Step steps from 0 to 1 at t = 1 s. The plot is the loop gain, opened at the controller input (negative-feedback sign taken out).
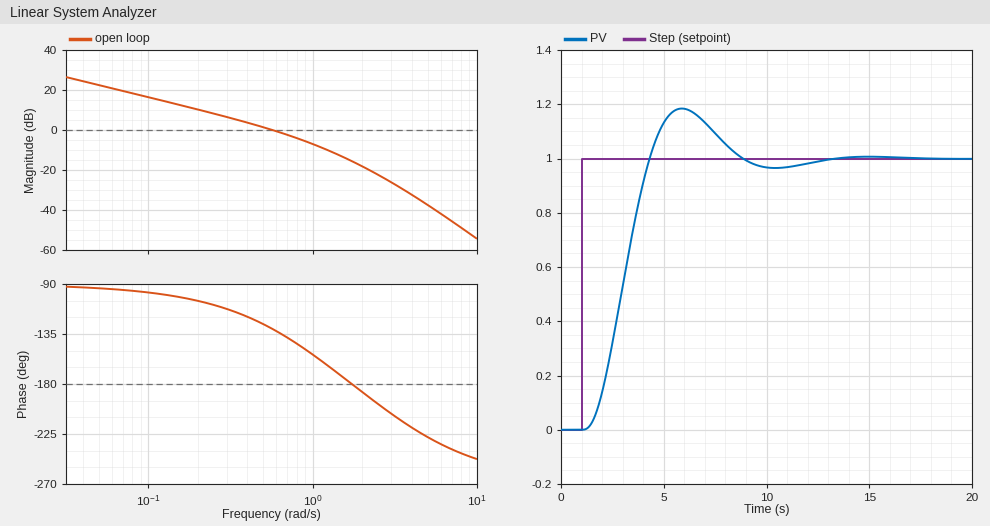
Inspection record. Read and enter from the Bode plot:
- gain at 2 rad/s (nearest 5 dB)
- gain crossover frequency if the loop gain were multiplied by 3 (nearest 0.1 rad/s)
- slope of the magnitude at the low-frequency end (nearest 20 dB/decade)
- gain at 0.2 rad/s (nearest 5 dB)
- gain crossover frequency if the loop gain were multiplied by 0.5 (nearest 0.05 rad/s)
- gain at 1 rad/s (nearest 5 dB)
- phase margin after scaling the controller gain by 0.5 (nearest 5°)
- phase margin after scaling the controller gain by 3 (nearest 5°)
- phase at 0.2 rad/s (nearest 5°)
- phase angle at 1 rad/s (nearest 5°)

-20 dB
1.2 rad/s
-20 dB/decade
10 dB
0.30 rad/s
-5 dB
65°
20°
-105°
-155°
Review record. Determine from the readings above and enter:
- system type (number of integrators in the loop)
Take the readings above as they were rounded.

1
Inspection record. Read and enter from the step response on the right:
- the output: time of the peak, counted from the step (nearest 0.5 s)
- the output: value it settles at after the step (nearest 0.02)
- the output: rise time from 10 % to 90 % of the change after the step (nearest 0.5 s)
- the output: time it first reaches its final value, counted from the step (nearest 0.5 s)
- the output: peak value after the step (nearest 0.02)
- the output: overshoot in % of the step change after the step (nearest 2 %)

5.0 s
1.00
2.0 s
3.5 s
1.18
18 %
